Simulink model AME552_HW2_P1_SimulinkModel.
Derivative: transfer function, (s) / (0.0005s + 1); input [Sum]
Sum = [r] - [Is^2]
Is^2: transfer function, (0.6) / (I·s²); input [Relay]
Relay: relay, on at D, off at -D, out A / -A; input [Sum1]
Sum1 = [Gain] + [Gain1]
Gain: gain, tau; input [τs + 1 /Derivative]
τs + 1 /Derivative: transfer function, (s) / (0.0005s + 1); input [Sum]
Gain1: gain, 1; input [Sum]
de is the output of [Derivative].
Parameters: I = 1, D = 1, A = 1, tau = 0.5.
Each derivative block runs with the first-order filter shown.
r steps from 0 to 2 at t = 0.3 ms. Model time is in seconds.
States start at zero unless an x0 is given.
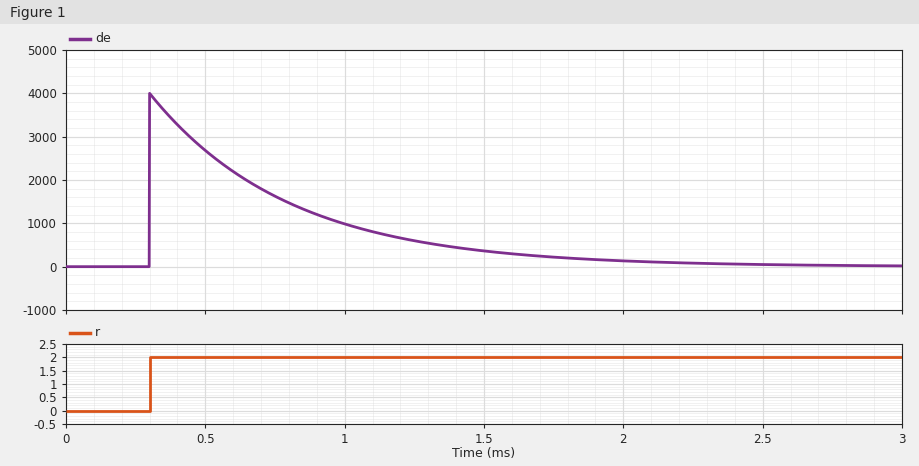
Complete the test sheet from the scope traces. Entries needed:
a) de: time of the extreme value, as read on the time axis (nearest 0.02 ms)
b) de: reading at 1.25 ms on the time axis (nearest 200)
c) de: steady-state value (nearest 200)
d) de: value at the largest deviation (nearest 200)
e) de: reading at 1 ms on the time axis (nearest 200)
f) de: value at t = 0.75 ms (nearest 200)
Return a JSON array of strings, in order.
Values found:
["0.30 ms", "600", "0", "4000", "1000", "1600"]
